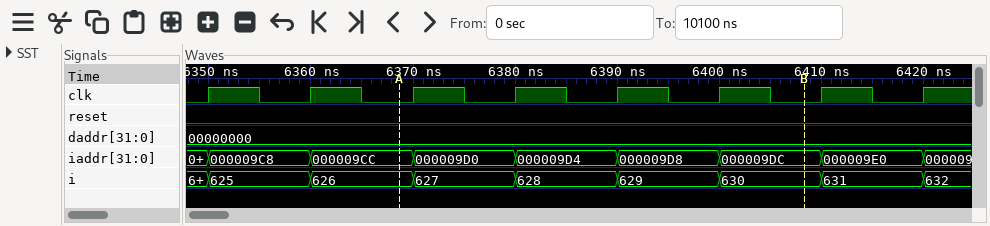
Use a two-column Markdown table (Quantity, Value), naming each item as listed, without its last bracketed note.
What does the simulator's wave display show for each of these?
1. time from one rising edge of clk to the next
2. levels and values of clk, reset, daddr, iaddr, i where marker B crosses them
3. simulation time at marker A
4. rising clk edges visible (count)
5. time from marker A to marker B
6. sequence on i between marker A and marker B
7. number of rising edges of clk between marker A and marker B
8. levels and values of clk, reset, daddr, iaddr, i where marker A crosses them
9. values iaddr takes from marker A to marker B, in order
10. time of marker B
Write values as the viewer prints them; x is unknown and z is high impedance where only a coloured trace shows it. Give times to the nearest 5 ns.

| Quantity | Value |
|---|---|
| time from one rising edge of clk to the next | 10 ns |
| levels and values of clk, reset, daddr, iaddr, i where marker B crosses them | clk=0, reset=0, daddr=00000000, iaddr=000009DC, i=630 |
| simulation time at marker A | 6370 ns |
| rising clk edges visible | 8 |
| time from marker A to marker B | 40 ns |
| sequence on i between marker A and marker B | 626, 627, 628, 629, 630 |
| number of rising edges of clk between marker A and marker B | 4 |
| levels and values of clk, reset, daddr, iaddr, i where marker A crosses them | clk=0, reset=0, daddr=00000000, iaddr=000009CC, i=626 |
| values iaddr takes from marker A to marker B, in order | 000009CC, 000009D0, 000009D4, 000009D8, 000009DC |
| time of marker B | 6410 ns |
